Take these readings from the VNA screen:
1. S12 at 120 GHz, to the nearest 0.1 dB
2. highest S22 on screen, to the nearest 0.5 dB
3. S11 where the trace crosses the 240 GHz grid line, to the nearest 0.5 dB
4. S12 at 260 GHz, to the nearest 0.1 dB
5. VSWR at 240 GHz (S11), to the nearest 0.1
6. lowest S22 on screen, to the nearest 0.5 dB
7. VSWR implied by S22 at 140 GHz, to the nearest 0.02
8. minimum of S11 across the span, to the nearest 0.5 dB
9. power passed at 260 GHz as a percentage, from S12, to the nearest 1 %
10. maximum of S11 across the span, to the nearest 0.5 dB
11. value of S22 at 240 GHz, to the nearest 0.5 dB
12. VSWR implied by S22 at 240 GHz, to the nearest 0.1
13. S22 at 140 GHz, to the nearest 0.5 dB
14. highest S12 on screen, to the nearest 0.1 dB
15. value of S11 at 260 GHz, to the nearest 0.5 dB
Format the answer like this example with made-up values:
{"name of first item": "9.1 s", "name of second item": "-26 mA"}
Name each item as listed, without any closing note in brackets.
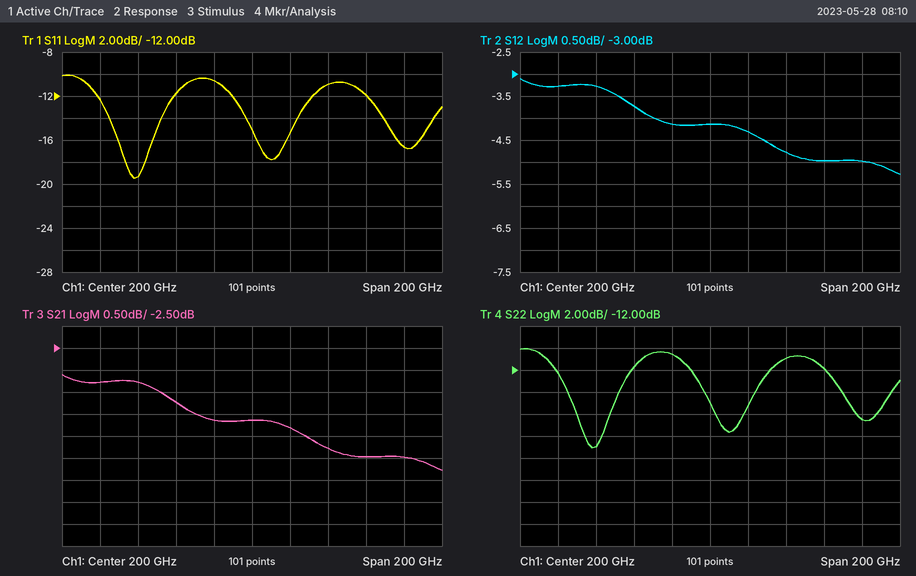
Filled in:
{"S12 at 120 GHz, to the nearest 0.1 dB": "-3.3 dB", "highest S22 on screen, to the nearest 0.5 dB": "-10.0 dB", "S11 where the trace crosses the 240 GHz grid line, to the nearest 0.5 dB": "-11.0 dB", "S12 at 260 GHz, to the nearest 0.1 dB": "-5.0 dB", "VSWR at 240 GHz (S11), to the nearest 0.1": "1.8", "lowest S22 on screen, to the nearest 0.5 dB": "-19.0 dB", "VSWR implied by S22 at 140 GHz, to the nearest 0.02": "1.26", "minimum of S11 across the span, to the nearest 0.5 dB": "-19.5 dB", "power passed at 260 GHz as a percentage, from S12, to the nearest 1 %": "32 %", "maximum of S11 across the span, to the nearest 0.5 dB": "-10.0 dB", "value of S22 at 240 GHz, to the nearest 0.5 dB": "-11.0 dB", "VSWR implied by S22 at 240 GHz, to the nearest 0.1": "1.8", "S22 at 140 GHz, to the nearest 0.5 dB": "-19.0 dB", "highest S12 on screen, to the nearest 0.1 dB": "-3.1 dB", "value of S11 at 260 GHz, to the nearest 0.5 dB": "-12.0 dB"}
